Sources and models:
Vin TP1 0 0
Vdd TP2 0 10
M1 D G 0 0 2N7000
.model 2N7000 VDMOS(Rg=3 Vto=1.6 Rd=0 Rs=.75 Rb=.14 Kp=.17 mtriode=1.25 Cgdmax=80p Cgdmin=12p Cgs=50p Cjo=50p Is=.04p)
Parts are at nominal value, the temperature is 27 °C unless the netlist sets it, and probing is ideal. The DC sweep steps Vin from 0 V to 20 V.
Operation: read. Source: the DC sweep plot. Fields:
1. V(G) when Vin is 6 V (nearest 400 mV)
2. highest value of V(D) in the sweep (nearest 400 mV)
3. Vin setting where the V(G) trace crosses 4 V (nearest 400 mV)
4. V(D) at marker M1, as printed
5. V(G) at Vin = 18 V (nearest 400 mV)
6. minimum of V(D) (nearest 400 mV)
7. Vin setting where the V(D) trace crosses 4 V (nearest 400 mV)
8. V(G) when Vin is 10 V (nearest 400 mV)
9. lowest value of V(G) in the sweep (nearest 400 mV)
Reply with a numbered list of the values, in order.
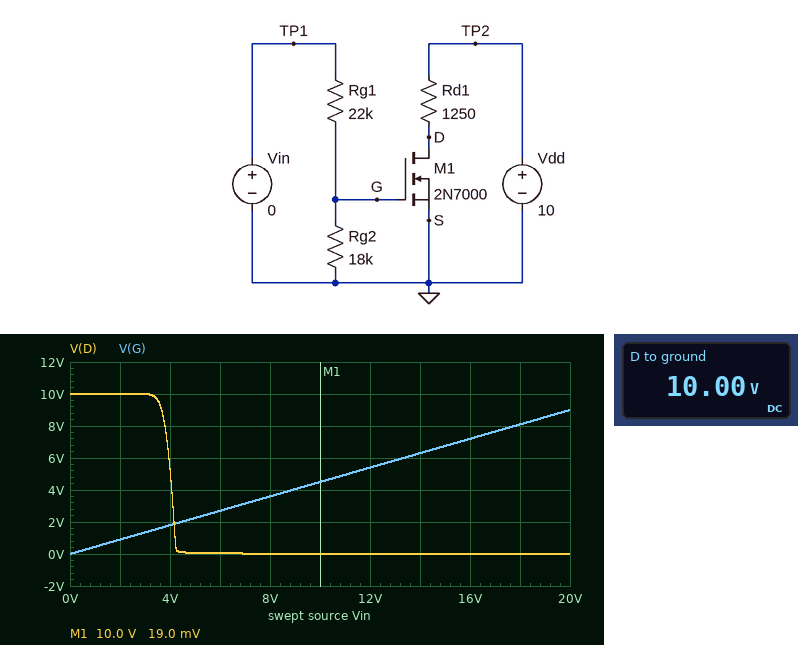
1. 2.8 V
2. 10.0 V
3. 8.8 V
4. 19.0 mV
5. 8.0 V
6. 0 V
7. 4.0 V
8. 4.4 V
9. 0 V
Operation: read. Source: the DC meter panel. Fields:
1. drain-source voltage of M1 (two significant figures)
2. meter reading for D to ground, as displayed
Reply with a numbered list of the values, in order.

1. 10 V
2. 10.00 V
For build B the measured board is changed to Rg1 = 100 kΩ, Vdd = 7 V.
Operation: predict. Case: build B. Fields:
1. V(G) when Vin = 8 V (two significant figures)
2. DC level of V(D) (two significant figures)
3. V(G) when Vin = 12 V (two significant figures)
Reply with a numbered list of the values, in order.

1. 1.2 V
2. 7.0 V
3. 1.8 V
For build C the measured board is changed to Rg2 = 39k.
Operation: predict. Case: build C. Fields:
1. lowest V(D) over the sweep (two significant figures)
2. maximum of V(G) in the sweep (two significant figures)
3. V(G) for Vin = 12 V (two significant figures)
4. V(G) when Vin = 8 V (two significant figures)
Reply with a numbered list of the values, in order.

1. 9.4 mV
2. 13 V
3. 7.7 V
4. 5.1 V
